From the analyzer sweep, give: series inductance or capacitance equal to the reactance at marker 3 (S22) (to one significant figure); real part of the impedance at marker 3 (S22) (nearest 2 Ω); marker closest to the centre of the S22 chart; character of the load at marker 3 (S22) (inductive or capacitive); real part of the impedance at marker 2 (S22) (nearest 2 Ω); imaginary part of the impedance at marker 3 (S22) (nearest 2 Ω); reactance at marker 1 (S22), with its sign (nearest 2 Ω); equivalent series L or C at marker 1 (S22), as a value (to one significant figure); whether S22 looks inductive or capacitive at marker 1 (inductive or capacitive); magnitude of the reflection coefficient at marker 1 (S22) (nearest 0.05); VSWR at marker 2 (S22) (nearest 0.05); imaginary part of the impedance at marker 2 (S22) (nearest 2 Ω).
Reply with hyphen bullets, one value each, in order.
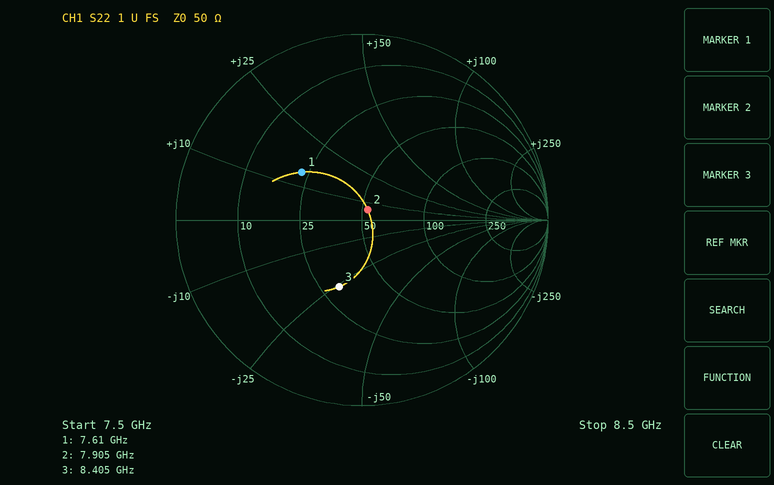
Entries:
- 700 fF
- 30 Ω
- marker 2
- capacitive
- 52 Ω
- -26 Ω
- +14 Ω
- 300 pH
- inductive
- 0.40
- 1.15
- +6 Ω
